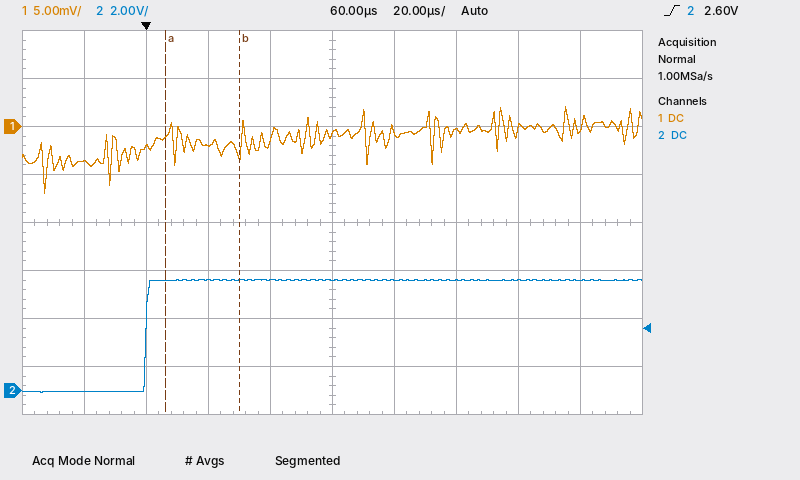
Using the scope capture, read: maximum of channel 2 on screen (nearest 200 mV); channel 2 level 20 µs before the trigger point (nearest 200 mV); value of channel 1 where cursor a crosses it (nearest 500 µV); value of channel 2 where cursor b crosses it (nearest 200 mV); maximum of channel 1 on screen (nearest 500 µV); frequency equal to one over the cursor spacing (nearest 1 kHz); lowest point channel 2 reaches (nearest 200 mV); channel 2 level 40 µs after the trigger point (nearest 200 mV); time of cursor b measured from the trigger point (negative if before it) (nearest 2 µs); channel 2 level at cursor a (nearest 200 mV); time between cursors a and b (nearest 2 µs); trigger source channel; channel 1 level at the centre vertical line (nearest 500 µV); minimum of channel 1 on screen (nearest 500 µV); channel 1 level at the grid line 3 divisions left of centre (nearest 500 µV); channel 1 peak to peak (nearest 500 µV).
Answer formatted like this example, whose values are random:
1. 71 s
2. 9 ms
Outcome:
1. 4.6 V
2. 0.0 V
3. -1.0 mV
4. 4.6 V
5. 2.0 mV
6. 42 kHz
7. 0.0 V
8. 4.6 V
9. +30 µs
10. 4.6 V
11. 24 µs
12. channel 2
13. -1.0 mV
14. -7.0 mV
15. -2.0 mV
16. 9.0 mV
